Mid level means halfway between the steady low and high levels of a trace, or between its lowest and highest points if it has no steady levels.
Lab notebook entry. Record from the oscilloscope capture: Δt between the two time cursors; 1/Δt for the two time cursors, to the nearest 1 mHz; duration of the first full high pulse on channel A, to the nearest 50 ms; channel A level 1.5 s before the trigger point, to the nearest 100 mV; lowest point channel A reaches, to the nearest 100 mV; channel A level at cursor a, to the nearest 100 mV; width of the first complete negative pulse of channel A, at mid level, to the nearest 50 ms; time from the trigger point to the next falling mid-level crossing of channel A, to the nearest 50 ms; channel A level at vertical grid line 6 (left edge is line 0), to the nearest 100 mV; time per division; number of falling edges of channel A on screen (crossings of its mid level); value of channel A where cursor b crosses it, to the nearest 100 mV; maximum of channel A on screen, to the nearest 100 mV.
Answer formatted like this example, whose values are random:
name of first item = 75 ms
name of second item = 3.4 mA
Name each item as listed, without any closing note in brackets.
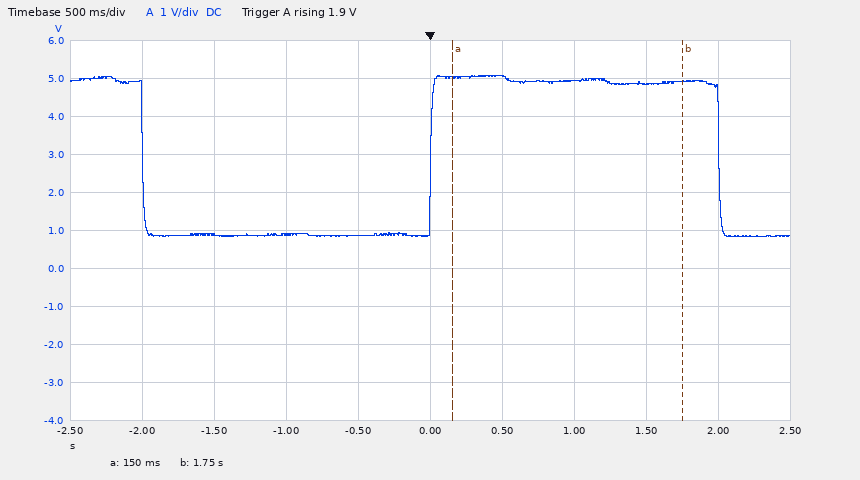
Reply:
Δt between the two time cursors = 1.60 s
1/Δt for the two time cursors, to the nearest 1 mHz = 625 mHz
duration of the first full high pulse on channel A, to the nearest 50 ms = 2.00 s
channel A level 1.5 s before the trigger point, to the nearest 100 mV = 900 mV
lowest point channel A reaches, to the nearest 100 mV = 800 mV
channel A level at cursor a, to the nearest 100 mV = 5.0 V
width of the first complete negative pulse of channel A, at mid level, to the nearest 50 ms = 2.00 s
time from the trigger point to the next falling mid-level crossing of channel A, to the nearest 50 ms = 2.00 s
channel A level at vertical grid line 6 (left edge is line 0), to the nearest 100 mV = 5.1 V
time per division = 500 ms
number of falling edges of channel A on screen = 2
value of channel A where cursor b crosses it, to the nearest 100 mV = 4.9 V
maximum of channel A on screen, to the nearest 100 mV = 5.1 V
